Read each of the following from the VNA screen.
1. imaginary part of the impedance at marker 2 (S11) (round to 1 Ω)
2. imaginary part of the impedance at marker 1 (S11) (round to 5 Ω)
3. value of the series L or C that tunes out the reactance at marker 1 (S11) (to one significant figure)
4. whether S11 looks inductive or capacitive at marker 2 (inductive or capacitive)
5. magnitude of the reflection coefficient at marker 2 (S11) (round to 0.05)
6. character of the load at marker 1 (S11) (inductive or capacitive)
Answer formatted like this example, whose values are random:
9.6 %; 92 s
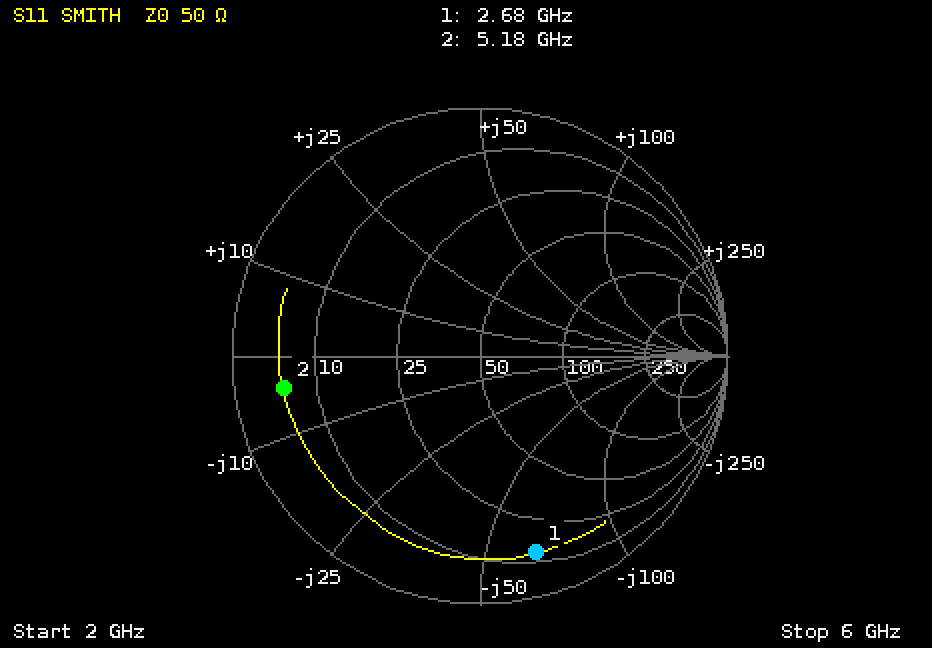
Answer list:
-4 Ω; -65 Ω; 4 nH; capacitive; 0.80; capacitive
